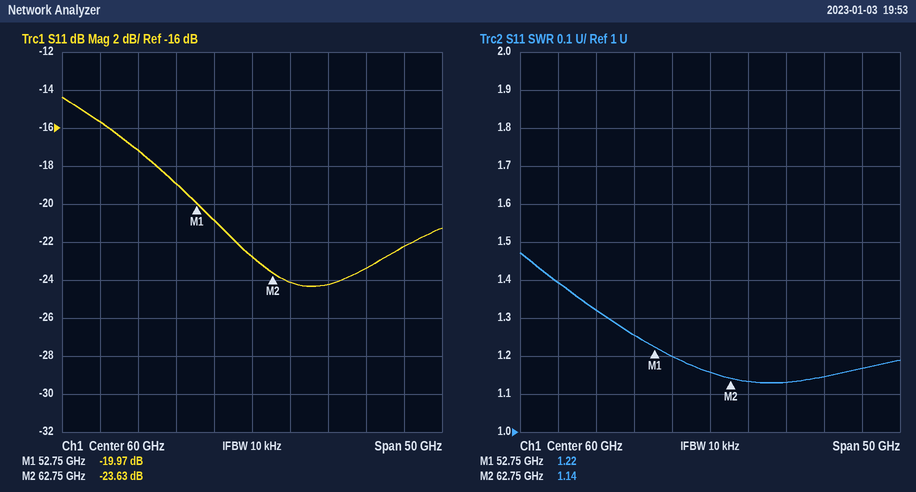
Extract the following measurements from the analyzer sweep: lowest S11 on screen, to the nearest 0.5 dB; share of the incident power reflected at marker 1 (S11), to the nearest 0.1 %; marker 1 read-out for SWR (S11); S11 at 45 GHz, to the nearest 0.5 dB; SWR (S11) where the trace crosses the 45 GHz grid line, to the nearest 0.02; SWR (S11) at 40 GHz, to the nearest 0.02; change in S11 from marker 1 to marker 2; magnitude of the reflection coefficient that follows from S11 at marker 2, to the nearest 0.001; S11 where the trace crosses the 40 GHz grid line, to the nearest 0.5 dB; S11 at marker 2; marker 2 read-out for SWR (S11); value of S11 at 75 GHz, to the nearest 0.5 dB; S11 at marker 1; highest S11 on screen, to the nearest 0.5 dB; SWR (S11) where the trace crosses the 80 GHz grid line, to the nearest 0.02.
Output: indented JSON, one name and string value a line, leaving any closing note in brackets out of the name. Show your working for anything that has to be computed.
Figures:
{
  "lowest S11 on screen, to the nearest 0.5 dB": "-24.5 dB",
  "share of the incident power reflected at marker 1 (S11), to the nearest 0.1 %": "10^(-19.97/10) ≈ 1.0 %",
  "marker 1 read-out for SWR": "1.22",
  "S11 at 45 GHz, to the nearest 0.5 dB": "-17.0 dB",
  "SWR (S11) where the trace crosses the 45 GHz grid line, to the nearest 0.02": "1.32",
  "SWR (S11) at 40 GHz, to the nearest 0.02": "1.40",
  "change in S11 from marker 1 to marker 2": "-23.63 − (-19.97) = -3.66 dB",
  "magnitude of the reflection coefficient that follows from S11 at marker 2, to the nearest 0.001": "10^(-23.63/20) ≈ 0.066",
  "S11 where the trace crosses the 40 GHz grid line, to the nearest 0.5 dB": "-15.5 dB",
  "S11 at marker 2": "-23.63 dB",
  "marker 2 read-out for SWR": "1.14",
  "value of S11 at 75 GHz, to the nearest 0.5 dB": "-23.5 dB",
  "S11 at marker 1": "-19.97 dB",
  "highest S11 on screen, to the nearest 0.5 dB": "-14.5 dB",
  "SWR (S11) where the trace crosses the 80 GHz grid line, to the nearest 0.02": "1.16"
}
